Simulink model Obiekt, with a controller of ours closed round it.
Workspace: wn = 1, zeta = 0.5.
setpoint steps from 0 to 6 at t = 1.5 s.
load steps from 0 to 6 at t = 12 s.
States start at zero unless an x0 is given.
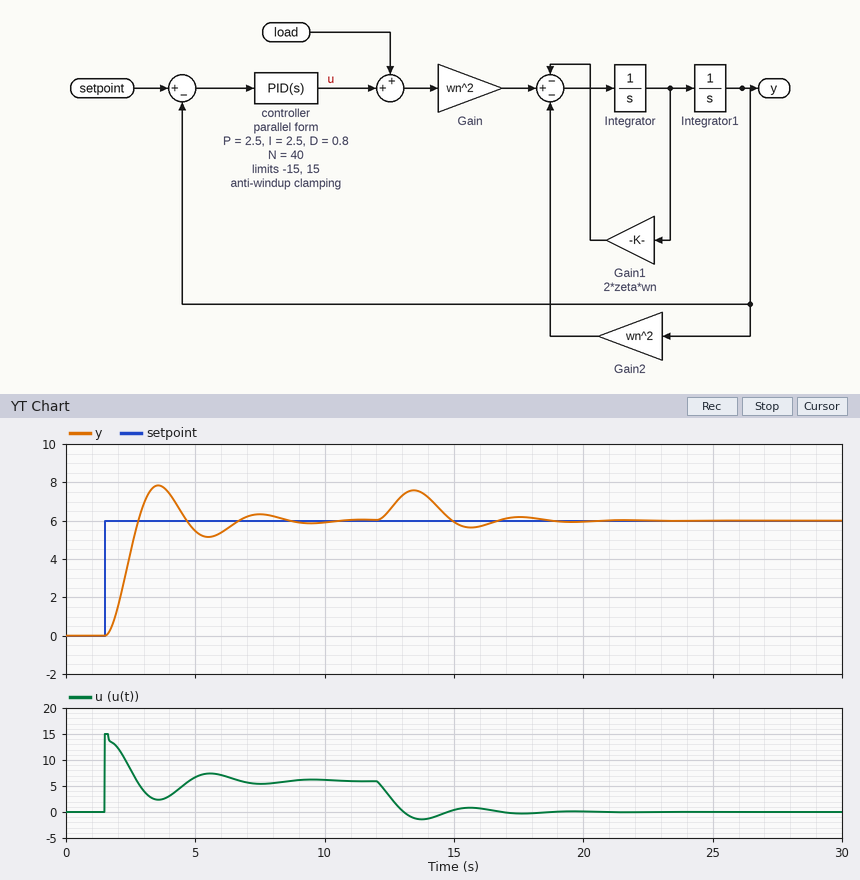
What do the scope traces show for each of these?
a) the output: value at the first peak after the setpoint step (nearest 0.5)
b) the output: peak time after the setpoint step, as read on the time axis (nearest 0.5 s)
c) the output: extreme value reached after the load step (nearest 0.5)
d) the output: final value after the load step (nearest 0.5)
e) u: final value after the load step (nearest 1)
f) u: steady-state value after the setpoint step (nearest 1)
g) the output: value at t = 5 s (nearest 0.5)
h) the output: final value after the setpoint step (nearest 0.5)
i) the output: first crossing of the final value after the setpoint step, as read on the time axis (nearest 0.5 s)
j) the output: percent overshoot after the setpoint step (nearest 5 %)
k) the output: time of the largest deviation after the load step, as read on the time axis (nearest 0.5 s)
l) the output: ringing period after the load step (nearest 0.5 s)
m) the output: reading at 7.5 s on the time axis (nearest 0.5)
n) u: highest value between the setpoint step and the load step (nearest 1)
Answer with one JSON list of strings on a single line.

["8.0", "3.5 s", "7.5", "6.0", "0", "6", "5.5", "6.0", "3.0 s", "30 %", "13.5 s", "4.0 s", "6.5", "15"]
